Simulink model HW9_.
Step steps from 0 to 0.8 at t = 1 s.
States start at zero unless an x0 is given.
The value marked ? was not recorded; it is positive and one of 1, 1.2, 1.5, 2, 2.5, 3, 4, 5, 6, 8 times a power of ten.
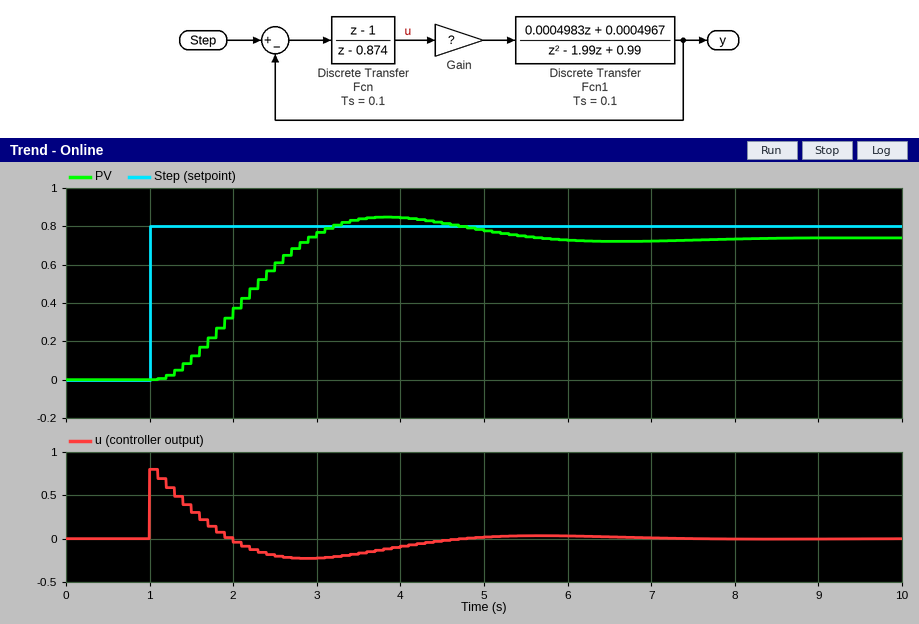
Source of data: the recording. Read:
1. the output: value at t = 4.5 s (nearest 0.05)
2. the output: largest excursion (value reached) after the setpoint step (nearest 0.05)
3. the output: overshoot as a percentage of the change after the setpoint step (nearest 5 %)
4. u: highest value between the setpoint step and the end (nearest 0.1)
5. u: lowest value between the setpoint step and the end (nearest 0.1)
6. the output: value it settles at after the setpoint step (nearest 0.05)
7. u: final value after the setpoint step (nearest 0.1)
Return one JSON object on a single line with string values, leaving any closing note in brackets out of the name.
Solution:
{"the output: value at t = 4.5 s": "0.80", "the output: largest excursion (value reached) after the setpoint step": "0.85", "the output: overshoot as a percentage of the change after the setpoint step": "15 %", "u: highest value between the setpoint step and the end": "0.8", "u: lowest value between the setpoint step and the end": "-0.2", "the output: value it settles at after the setpoint step": "0.75", "u: final value after the setpoint step": "0.0"}
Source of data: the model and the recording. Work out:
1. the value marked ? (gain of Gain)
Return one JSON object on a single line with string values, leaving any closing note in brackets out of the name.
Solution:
{"the value marked ?": "15"}
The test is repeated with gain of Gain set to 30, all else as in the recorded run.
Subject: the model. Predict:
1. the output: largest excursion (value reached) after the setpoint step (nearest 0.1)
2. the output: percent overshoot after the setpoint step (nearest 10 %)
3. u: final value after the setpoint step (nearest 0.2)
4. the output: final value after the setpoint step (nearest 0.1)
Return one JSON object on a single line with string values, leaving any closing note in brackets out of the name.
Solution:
{"the output: largest excursion (value reached) after the setpoint step": "1.0", "the output: percent overshoot after the setpoint step": "30 %", "u: final value after the setpoint step": "0.0", "the output: final value after the setpoint step": "0.8"}
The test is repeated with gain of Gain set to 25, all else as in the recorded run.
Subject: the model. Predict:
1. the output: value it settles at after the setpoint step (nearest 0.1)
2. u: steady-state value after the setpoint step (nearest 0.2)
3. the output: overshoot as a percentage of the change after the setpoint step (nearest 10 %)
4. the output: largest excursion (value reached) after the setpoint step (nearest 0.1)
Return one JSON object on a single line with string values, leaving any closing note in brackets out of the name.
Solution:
{"the output: value it settles at after the setpoint step": "0.8", "u: steady-state value after the setpoint step": "0.0", "the output: overshoot as a percentage of the change after the setpoint step": "30 %", "the output: largest excursion (value reached) after the setpoint step": "1.0"}
